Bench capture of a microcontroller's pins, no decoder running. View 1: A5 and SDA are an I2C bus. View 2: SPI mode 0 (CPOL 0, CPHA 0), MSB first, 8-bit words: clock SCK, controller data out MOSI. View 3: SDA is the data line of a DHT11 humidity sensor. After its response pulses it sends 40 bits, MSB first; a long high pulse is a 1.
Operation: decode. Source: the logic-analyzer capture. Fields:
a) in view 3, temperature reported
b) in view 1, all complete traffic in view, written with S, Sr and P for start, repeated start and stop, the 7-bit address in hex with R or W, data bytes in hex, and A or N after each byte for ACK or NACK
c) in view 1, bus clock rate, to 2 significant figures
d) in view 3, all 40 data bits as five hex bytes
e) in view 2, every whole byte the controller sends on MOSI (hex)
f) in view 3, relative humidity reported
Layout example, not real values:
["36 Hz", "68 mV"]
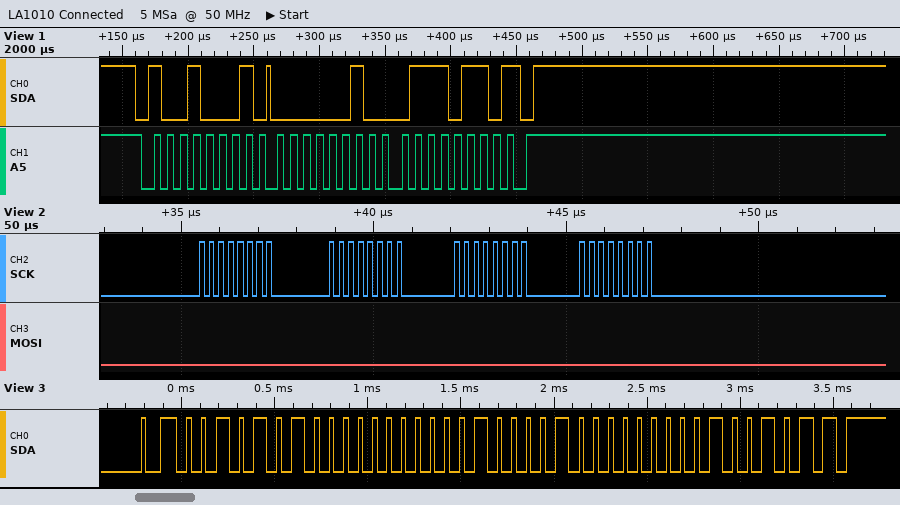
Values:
["33.0 °C", "S 48R A 02 A 76 N P", "100 kHz", "2A 00 21 00 4B", "00 00 00 00", "42 %"]
